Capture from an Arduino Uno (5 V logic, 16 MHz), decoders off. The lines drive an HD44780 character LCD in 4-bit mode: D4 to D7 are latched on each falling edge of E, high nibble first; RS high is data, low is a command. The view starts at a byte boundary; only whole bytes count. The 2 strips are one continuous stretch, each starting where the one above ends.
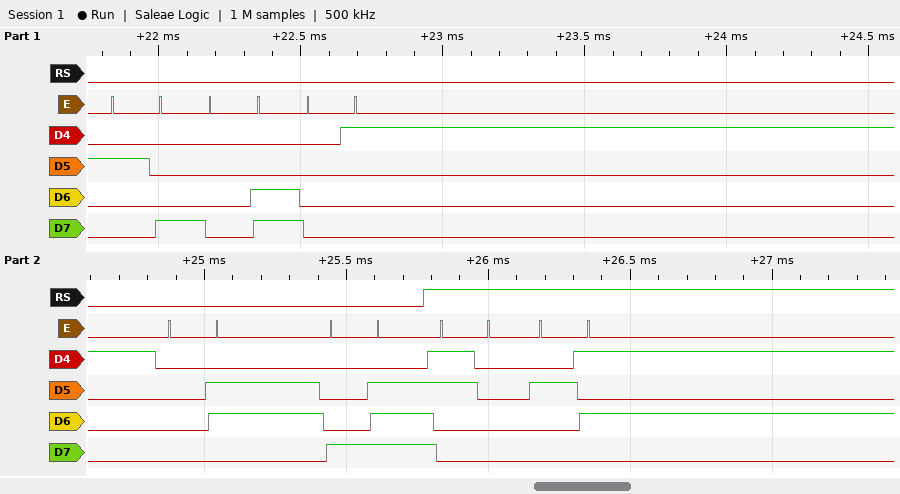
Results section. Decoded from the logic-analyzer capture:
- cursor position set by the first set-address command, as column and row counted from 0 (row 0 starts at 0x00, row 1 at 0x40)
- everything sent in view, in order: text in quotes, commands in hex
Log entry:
column 14, row 0
0x28 0x0C 0x01 0x06 0x8E "0%"
